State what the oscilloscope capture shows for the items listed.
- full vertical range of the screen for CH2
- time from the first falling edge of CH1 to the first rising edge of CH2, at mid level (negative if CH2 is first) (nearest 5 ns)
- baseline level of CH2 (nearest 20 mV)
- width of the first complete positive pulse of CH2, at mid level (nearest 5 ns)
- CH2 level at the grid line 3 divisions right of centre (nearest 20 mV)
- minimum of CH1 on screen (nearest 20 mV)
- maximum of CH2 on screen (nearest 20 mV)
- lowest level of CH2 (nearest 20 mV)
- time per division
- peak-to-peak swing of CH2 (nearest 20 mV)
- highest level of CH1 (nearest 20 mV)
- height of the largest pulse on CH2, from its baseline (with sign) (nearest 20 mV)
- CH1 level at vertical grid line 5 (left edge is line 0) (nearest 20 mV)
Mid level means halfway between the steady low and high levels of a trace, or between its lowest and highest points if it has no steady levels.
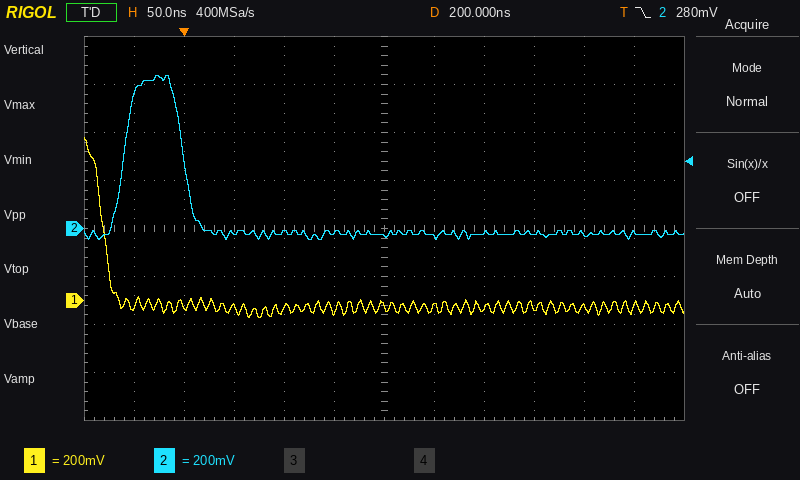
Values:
1.6 V
+20 ns
-20 mV
60 ns
-20 mV
-80 mV
640 mV
-40 mV
50 ns
680 mV
680 mV
+660 mV
-40 mV
